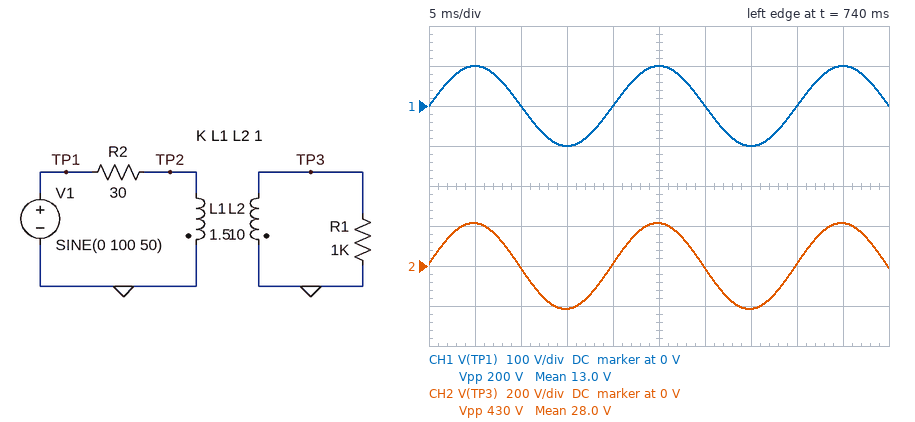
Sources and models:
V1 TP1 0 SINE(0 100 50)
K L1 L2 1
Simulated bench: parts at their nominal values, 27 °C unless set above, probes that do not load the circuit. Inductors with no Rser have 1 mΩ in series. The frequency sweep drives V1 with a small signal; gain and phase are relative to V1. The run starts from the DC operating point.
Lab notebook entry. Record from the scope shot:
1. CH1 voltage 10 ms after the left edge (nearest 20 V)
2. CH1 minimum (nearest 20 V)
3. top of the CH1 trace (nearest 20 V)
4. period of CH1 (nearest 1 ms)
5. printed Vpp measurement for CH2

0 V
-100 V
100 V
20 ms
430 V
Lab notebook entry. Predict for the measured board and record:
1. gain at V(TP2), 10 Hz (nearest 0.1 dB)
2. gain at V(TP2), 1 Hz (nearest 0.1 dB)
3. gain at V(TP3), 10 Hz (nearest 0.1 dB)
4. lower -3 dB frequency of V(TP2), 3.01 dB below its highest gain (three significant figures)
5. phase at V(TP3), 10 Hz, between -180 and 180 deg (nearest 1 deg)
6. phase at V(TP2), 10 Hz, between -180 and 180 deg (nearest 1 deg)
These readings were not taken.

-1.9 dB
-10.6 dB
6.4 dB
2.65 Hz
15 deg
15 deg
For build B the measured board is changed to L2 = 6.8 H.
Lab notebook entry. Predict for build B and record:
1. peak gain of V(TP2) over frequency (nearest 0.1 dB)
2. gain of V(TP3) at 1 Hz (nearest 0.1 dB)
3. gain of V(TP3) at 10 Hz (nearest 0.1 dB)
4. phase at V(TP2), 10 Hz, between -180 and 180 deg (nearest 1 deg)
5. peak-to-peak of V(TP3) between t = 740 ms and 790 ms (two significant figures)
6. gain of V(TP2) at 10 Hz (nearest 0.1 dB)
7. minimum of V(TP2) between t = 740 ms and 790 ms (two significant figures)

-1.1 dB
-4.0 dB
5.1 dB
16 deg
370 V
-1.4 dB
-88 V
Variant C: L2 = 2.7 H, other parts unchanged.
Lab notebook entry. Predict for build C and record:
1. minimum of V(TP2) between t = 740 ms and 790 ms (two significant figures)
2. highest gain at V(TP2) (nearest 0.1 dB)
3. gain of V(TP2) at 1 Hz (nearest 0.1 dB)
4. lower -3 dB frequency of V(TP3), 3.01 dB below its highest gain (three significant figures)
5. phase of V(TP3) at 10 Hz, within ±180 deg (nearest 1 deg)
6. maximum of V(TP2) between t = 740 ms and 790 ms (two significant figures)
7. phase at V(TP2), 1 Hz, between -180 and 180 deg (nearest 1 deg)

-95 V
-0.5 dB
-10.5 dB
3.02 Hz
17 deg
95 V
72 deg
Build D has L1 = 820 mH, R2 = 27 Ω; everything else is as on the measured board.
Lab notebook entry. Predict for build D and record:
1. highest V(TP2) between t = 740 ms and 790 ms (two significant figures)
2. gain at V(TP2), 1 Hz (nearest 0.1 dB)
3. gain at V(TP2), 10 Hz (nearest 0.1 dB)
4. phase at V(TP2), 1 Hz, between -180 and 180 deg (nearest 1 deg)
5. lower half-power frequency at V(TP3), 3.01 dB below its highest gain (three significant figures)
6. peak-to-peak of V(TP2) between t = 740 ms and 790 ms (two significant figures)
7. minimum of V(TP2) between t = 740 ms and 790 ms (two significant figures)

75 V
-14.7 dB
-3.1 dB
76 deg
3.94 Hz
150 V
-75 V
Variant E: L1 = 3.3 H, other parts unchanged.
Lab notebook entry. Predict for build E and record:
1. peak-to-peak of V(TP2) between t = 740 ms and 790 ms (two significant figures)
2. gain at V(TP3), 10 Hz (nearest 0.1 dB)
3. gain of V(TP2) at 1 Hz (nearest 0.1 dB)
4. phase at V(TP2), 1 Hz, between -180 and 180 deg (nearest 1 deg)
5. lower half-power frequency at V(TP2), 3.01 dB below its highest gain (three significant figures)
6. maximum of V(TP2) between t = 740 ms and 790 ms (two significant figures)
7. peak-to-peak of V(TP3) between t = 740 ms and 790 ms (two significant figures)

180 V
4.0 dB
-5.2 dB
53 deg
1.33 Hz
92 V
320 V
